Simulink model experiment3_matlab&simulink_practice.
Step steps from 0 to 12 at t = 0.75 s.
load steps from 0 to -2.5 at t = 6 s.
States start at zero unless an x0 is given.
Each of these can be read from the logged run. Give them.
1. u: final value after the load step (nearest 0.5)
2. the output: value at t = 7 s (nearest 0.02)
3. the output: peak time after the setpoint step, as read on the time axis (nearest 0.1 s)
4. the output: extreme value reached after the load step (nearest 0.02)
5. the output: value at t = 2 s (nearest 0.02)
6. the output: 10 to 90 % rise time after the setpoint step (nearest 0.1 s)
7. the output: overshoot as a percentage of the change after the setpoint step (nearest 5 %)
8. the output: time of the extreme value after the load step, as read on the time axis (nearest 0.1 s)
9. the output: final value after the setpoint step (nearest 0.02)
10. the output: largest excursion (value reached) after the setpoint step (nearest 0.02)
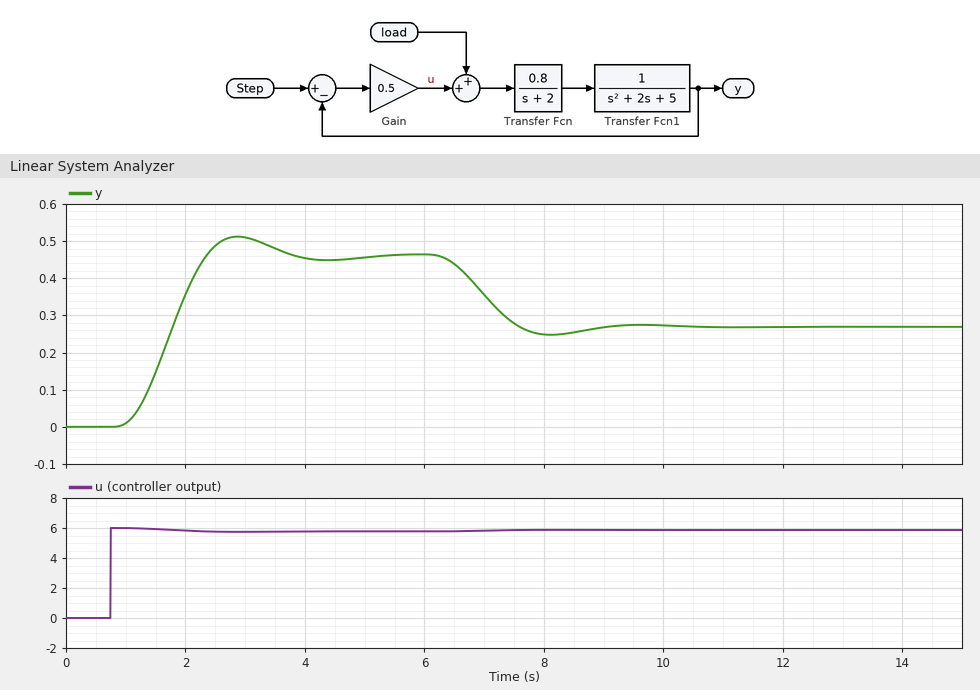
6.0
0.36
2.9 s
0.24
0.36
1.0 s
10 %
8.1 s
0.46
0.52
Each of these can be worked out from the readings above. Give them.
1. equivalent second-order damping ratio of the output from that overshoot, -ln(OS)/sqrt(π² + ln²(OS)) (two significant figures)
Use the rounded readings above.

0.59
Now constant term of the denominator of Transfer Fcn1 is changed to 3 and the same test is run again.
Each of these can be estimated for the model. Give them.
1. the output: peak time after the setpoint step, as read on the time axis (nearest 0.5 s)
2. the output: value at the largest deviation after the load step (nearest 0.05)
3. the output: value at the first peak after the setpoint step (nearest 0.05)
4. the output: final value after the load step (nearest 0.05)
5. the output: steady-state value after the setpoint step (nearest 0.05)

3.5 s
0.40
0.80
0.45
0.75
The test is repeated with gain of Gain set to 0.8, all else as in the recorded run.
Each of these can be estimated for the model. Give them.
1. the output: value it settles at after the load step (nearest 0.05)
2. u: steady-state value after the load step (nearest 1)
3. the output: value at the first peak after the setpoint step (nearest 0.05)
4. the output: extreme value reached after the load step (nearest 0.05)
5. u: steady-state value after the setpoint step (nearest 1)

0.55
9
0.80
0.50
9
